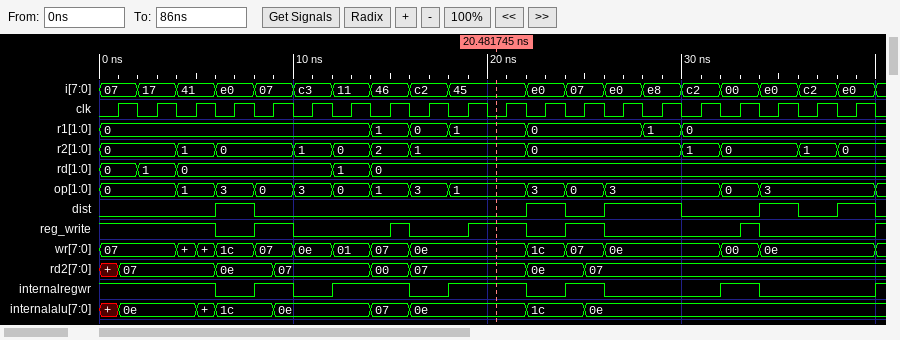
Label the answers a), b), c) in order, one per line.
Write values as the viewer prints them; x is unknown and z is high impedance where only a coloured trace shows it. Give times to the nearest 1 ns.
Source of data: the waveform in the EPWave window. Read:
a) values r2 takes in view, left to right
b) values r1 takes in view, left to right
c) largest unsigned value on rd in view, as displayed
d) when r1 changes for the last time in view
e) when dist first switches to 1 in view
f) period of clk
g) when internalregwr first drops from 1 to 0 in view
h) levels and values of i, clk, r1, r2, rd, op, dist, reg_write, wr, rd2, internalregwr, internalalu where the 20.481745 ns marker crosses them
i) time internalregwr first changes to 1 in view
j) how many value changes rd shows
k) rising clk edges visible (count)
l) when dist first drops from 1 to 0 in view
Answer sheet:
a) 0, 1, 0, 1, 0, 2, 1, 0, 1, 0, 1, 0
b) 0, 1, 0, 1, 0, 1, 0
c) 1
d) 30 ns
e) 6 ns
f) 2 ns
g) 6 ns
h) i=45, clk=0, r1=1, r2=1, rd=0, op=1, dist=0, reg_write=1, wr=0e, rd2=07, internalregwr=1, internalalu=0e
i) 8 ns
j) 4
k) 20
l) 8 ns
